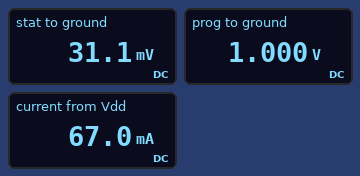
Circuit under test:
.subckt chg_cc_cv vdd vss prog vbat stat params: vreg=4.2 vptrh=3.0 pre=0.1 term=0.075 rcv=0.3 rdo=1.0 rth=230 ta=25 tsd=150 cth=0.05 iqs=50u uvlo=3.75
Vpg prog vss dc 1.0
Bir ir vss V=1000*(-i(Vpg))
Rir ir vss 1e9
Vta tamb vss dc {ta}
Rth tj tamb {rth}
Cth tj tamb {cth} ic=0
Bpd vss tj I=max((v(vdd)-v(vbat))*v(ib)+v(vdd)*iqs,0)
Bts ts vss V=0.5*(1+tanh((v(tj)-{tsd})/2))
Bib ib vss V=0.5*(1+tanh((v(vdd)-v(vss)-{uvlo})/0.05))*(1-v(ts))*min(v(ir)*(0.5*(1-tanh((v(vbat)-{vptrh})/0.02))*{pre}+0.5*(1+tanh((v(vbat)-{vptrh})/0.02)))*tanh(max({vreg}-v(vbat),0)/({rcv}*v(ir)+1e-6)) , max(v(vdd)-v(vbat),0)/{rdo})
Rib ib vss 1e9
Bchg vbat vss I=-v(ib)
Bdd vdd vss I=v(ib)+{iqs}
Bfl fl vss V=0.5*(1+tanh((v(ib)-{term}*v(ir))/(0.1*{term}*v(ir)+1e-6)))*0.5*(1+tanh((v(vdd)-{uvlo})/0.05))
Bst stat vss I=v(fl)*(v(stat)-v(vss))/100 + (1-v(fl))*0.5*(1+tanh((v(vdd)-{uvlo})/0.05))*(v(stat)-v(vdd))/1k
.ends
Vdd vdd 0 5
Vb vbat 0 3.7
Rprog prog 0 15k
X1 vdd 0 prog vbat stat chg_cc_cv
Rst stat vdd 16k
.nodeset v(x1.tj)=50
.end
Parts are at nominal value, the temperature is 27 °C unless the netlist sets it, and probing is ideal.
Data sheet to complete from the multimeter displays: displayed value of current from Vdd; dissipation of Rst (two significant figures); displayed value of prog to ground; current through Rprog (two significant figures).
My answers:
67.0 mA
1.5 mW
1.000 V
67 µA
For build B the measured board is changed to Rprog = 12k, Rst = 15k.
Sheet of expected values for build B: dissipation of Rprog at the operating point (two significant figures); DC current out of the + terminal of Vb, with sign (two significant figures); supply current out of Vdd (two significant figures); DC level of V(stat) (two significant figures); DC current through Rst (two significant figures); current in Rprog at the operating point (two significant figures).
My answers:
83 µW
-83 mA
84 mA
33 mV
330 µA
83 µA
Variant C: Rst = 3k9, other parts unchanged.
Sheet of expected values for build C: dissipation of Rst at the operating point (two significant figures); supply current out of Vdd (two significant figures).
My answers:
6.1 mW
68 mA
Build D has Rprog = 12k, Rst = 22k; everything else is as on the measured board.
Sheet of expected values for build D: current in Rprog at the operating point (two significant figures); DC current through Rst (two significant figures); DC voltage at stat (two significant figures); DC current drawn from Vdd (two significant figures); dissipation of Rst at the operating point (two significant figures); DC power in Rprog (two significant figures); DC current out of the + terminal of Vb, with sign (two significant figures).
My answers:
83 µA
230 µA
23 mV
84 mA
1.1 mW
83 µW
-83 mA
